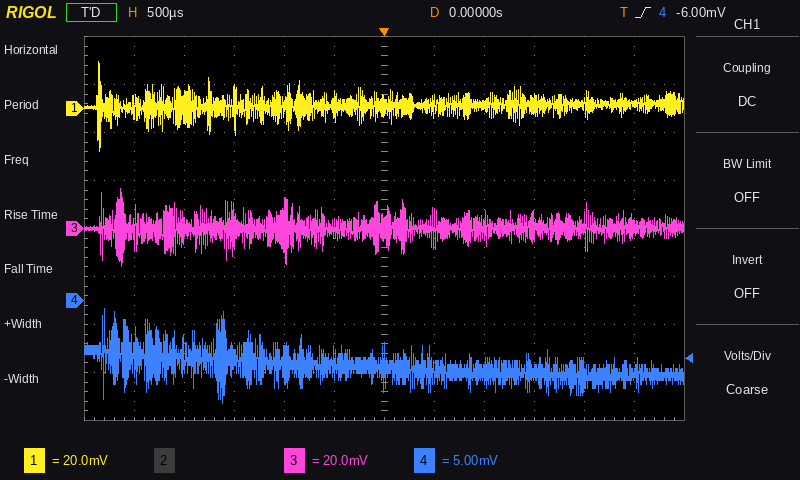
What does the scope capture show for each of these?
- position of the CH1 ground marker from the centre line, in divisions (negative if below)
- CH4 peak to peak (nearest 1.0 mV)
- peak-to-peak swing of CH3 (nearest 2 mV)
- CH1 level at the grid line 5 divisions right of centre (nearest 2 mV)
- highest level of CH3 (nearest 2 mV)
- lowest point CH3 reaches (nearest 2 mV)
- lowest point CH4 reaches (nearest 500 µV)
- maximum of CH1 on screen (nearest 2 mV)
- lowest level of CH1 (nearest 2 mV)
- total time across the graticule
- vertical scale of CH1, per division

+2.5 div
10.0 mV
32 mV
2 mV
16 mV
-16 mV
-10.5 mV
20 mV
-18 mV
6 ms
20 mV
